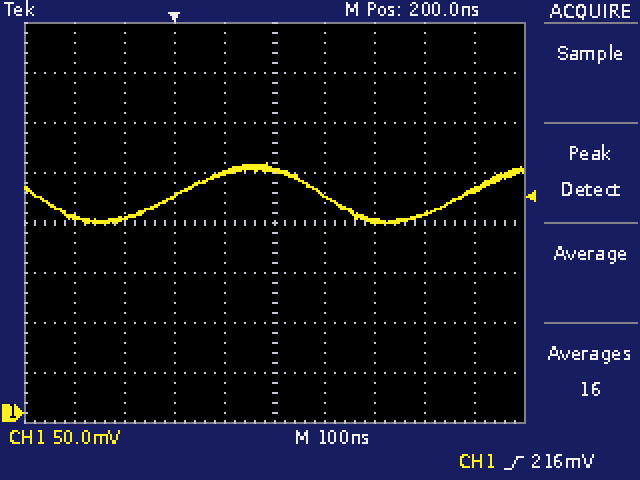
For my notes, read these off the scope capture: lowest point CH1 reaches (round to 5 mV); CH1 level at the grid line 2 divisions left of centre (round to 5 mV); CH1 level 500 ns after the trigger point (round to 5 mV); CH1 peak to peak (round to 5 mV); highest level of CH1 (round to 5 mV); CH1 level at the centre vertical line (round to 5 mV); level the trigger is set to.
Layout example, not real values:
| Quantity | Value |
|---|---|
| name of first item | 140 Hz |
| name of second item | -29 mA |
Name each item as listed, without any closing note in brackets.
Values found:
| Quantity | Value |
|---|---|
| lowest point CH1 reaches | 190 mV |
| CH1 level at the grid line 2 divisions left of centre | 215 mV |
| CH1 level 500 ns after the trigger point | 200 mV |
| CH1 peak to peak | 60 mV |
| highest level of CH1 | 250 mV |
| CH1 level at the centre vertical line | 245 mV |
| level the trigger is set to | 216 mV |
